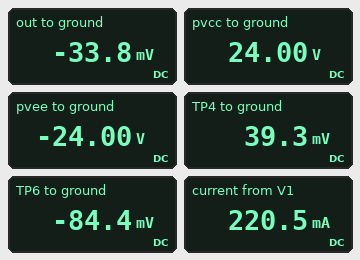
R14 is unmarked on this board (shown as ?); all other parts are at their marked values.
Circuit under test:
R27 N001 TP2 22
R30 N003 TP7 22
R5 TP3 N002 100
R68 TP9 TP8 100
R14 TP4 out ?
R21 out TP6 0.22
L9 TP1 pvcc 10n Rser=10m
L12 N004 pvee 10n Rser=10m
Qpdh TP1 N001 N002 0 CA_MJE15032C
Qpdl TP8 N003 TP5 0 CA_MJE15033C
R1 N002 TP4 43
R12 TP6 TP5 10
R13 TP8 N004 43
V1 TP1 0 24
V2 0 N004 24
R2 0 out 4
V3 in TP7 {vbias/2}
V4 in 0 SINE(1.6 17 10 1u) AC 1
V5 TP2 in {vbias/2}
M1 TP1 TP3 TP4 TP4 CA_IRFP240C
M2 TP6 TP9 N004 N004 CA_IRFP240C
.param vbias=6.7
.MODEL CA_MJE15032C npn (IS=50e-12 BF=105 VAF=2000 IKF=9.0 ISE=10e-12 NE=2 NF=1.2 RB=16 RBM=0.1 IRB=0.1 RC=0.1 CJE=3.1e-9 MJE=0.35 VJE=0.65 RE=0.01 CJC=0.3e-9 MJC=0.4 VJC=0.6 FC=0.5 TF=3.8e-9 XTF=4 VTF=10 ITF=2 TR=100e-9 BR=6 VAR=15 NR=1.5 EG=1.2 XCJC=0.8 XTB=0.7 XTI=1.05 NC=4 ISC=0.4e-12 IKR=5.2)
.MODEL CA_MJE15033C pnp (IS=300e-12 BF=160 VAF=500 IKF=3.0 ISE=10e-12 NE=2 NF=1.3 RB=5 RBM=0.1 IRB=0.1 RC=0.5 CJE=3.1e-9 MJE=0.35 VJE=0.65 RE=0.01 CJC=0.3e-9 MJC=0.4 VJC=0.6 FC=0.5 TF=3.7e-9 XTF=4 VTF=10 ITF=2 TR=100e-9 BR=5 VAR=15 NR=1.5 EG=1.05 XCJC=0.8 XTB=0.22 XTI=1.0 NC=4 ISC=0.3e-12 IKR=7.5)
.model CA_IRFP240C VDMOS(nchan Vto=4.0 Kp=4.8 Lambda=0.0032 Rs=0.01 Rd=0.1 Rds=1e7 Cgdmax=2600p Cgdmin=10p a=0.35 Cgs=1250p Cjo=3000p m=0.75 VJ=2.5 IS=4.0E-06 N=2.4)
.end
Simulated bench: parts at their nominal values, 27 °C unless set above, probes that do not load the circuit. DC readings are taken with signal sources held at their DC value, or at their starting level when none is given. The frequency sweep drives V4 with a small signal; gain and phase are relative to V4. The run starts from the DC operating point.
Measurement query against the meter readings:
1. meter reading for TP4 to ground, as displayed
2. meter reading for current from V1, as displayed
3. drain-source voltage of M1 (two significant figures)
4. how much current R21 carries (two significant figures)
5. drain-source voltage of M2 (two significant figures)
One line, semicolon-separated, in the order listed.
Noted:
39.3 mV; 220.5 mA; 24 V; 230 mA; 24 V
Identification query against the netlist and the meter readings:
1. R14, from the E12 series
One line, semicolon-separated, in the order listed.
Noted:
0.33 Ω
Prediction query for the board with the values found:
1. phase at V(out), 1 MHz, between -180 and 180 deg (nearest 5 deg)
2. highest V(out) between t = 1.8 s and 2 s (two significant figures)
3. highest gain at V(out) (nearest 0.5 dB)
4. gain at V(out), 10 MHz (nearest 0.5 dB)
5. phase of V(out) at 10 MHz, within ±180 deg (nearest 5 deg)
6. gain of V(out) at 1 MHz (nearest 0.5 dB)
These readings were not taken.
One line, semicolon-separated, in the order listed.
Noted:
-5 deg; 15 V; 0 dB; -5.0 dB; -105 deg; -0.5 dB
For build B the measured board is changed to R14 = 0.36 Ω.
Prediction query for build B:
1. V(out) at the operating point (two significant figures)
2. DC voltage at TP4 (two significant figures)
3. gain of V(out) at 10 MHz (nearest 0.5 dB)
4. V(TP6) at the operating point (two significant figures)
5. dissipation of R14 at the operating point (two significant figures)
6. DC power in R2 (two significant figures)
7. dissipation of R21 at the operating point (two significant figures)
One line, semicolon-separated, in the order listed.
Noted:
-35 mV; 43 mV; -5.5 dB; -85 mV; 17 mW; 310 µW; 11 mW
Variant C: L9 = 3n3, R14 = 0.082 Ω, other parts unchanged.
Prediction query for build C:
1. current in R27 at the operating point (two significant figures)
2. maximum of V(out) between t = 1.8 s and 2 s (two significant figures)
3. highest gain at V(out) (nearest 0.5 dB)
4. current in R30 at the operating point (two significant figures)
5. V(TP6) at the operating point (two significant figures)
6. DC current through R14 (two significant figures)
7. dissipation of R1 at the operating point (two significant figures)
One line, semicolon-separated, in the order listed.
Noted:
980 µA; 16 V; 0.5 dB; 650 µA; -77 mV; 260 mA; 420 mW
